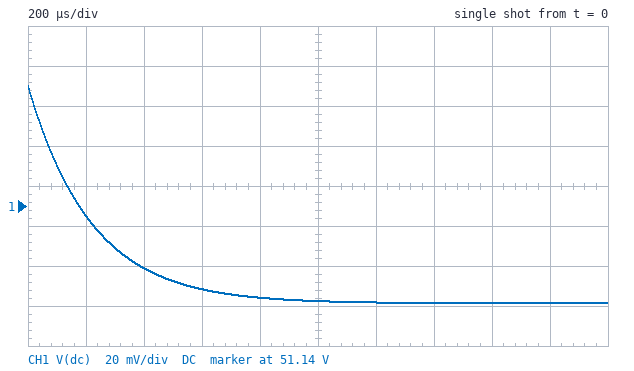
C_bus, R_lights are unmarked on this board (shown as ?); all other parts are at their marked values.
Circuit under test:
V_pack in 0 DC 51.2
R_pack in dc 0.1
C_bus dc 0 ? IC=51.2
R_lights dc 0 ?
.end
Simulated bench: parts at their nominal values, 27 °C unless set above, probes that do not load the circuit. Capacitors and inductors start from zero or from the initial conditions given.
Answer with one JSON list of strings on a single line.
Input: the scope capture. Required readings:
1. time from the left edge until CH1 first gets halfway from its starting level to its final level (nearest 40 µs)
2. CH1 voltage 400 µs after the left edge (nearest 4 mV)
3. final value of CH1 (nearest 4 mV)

["160 µs", "51.108 V", "51.092 V"]
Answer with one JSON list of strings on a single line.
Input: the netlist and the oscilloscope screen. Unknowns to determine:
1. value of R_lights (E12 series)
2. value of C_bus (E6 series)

["47 Ω", "2.2 mF"]
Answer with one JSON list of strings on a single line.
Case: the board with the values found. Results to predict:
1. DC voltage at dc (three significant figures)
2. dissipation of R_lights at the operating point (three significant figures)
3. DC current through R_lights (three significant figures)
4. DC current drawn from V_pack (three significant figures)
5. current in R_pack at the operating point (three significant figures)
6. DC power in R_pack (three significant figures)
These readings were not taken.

["51.1 V", "55.5 W", "1.09 A", "1.09 A", "1.09 A", "118 mW"]
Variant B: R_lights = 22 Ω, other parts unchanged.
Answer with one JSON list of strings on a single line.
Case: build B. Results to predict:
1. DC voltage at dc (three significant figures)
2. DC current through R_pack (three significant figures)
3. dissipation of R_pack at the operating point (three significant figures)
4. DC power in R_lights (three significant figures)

["51.0 V", "2.32 A", "537 mW", "118 W"]
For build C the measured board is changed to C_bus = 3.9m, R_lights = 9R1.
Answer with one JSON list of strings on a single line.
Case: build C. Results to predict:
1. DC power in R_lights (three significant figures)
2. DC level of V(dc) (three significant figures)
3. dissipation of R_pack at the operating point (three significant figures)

["282 W", "50.6 V", "3.10 W"]
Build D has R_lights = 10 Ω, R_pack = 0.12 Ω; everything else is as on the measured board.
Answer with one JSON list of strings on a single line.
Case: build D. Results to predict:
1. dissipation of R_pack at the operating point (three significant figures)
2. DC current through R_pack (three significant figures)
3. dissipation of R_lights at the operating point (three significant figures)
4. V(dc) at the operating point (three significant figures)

["3.07 W", "5.06 A", "256 W", "50.6 V"]
